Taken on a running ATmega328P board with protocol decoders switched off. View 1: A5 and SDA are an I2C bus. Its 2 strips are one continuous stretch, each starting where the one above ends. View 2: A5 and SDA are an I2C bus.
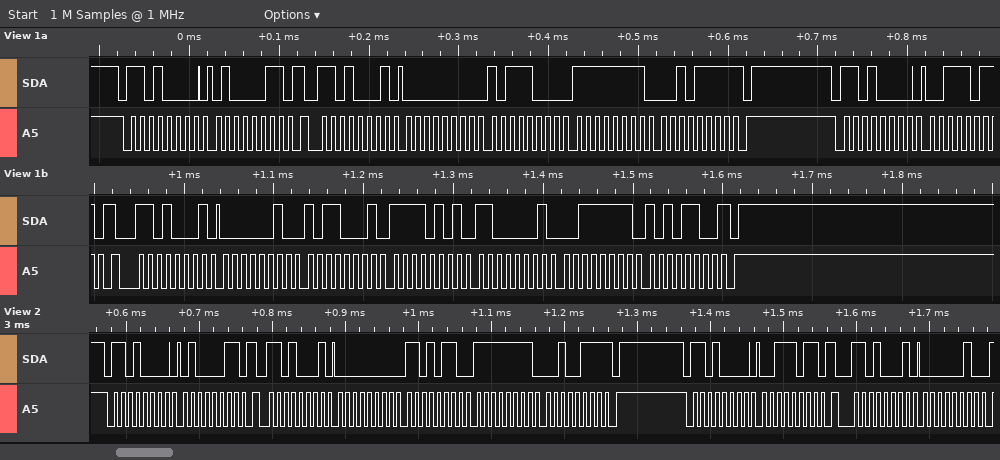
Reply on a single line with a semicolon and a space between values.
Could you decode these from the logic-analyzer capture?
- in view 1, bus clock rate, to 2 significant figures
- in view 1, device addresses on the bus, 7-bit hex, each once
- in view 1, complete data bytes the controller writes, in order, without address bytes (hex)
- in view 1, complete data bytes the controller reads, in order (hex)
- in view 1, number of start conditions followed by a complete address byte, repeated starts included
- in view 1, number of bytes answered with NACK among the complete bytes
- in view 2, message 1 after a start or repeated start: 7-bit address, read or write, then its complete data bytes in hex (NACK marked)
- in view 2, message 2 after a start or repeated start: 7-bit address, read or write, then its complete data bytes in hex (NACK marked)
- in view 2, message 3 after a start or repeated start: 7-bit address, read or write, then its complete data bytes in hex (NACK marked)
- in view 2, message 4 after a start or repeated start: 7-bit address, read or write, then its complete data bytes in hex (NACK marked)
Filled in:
100 kHz; 0x68; 43 3B; 00 B8 FF 2F 02 B1 F5 C1 3F AC; 4; 2; 0x68 write: 43; 0x68 read: 00 D6 FF 27 NACK; 0x68 write: 3B; 0x68 read: 02
